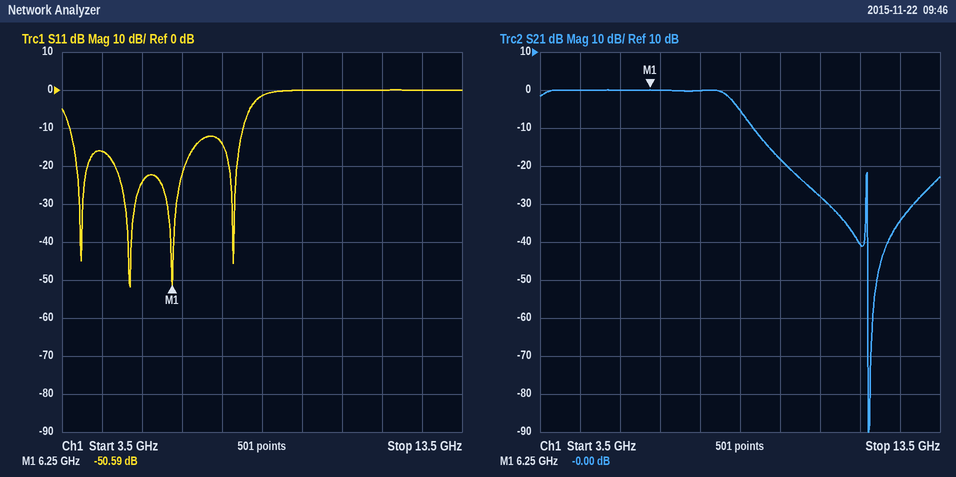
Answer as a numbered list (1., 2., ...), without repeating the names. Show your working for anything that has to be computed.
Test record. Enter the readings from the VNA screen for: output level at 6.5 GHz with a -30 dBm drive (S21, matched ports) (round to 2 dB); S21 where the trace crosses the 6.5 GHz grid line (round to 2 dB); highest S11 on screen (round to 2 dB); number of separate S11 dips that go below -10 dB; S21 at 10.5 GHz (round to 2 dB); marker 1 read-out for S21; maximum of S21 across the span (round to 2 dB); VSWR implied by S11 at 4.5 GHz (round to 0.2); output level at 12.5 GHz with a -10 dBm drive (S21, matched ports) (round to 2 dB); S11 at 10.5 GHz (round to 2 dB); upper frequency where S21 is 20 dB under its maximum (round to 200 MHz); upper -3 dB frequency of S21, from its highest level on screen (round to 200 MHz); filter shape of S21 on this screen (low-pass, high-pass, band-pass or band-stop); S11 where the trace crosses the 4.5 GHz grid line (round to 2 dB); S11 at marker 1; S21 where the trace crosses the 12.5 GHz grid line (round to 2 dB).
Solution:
1. -30 dBm + (0 dB) = -30 dBm
2. 0 dB
3. 0 dB
4. 4
5. -28 dB
6. -0.00 dB
7. 0 dB
8. |Γ| = 10^(-16/20) = 0.1585; VSWR = (1 + 0.1585)/(1 − 0.1585) ≈ 1.4
9. -10 dBm + (-34 dB) = -44 dBm
10. 0 dB
11. 9.6 GHz
12. 8.4 GHz
13. low-pass
14. -16 dB
15. -50.59 dB
16. -34 dB
